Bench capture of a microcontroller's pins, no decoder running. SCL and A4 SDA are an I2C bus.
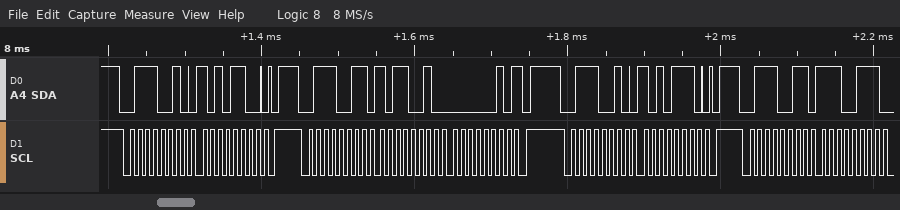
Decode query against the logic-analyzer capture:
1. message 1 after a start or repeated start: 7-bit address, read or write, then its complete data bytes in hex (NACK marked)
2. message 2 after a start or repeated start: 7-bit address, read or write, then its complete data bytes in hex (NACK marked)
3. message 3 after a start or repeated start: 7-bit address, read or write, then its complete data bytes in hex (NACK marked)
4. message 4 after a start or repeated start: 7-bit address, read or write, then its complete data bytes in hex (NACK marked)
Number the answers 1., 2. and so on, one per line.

1. 0x39 write: AC
2. 0x39 read: B2 02 NACK
3. 0x39 write: AE
4. 0x39 read: E7
